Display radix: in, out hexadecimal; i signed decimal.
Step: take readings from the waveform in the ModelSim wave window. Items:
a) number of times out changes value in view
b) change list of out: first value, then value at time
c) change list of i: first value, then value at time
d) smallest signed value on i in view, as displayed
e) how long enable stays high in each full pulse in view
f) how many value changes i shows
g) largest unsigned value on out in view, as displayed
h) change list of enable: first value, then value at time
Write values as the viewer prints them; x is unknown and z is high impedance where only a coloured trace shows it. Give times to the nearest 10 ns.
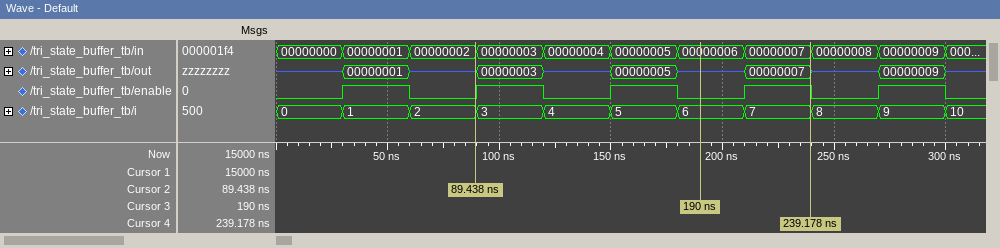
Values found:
10
z, 00000001 at 30 ns, z at 60 ns, 00000003 at 90 ns, z at 120 ns, 00000005 at 150 ns, z at 180 ns, 00000007 at 210 ns, z at 240 ns, 00000009 at 270 ns, z at 300 ns
0, 1 at 30 ns, 2 at 60 ns, 3 at 90 ns, 4 at 120 ns, 5 at 150 ns, 6 at 180 ns, 7 at 210 ns, 8 at 240 ns, 9 at 270 ns, 10 at 300 ns
0
30 ns, 30 ns, 30 ns, 30 ns, 30 ns
10
00000009
0, 1 at 30 ns, 0 at 60 ns, 1 at 90 ns, 0 at 120 ns, 1 at 150 ns, 0 at 180 ns, 1 at 210 ns, 0 at 240 ns, 1 at 270 ns, 0 at 300 ns
